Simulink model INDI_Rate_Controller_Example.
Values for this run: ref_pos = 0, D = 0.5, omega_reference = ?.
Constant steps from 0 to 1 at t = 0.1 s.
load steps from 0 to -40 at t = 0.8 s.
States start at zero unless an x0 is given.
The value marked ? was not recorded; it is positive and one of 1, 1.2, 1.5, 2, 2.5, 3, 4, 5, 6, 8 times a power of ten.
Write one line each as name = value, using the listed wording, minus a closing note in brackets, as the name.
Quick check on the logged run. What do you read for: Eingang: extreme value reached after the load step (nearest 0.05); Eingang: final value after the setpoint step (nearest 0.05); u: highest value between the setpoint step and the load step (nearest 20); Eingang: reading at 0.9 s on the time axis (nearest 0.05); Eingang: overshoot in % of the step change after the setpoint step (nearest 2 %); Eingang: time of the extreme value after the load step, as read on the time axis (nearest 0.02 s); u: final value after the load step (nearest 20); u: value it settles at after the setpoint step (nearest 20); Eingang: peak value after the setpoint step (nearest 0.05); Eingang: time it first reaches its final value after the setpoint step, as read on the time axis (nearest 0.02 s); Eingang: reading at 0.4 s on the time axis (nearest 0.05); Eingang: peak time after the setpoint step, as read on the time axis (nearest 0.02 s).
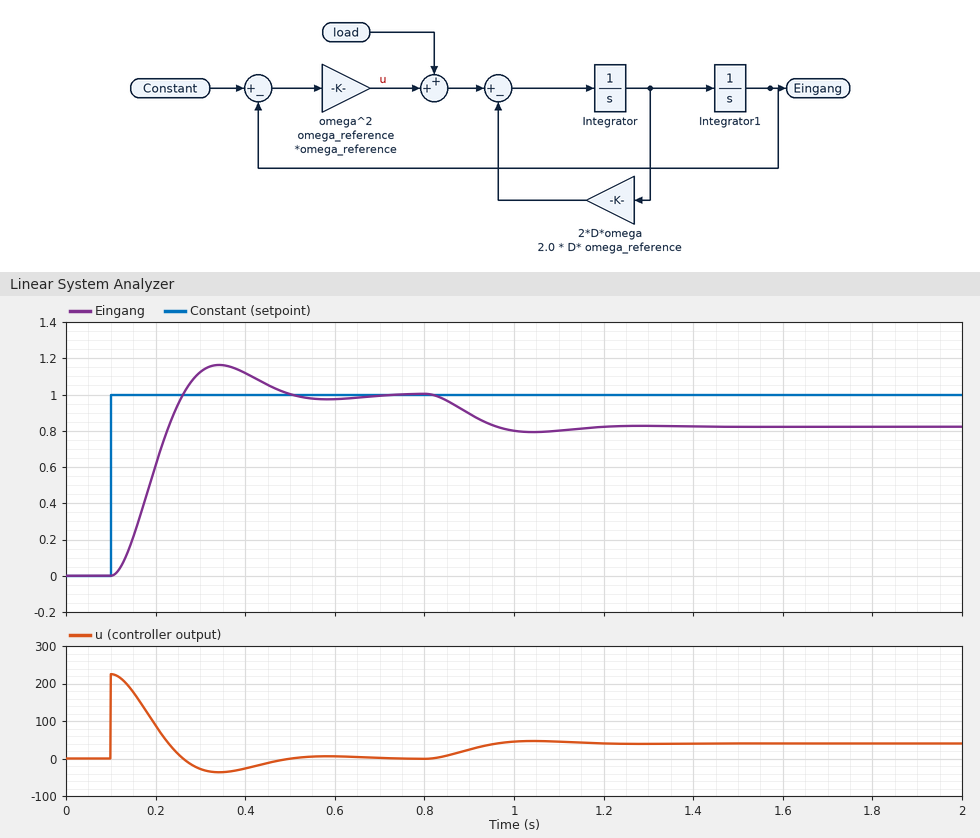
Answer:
Eingang: extreme value reached after the load step = 0.80
Eingang: final value after the setpoint step = 1.00
u: highest value between the setpoint step and the load step = 220
Eingang: reading at 0.9 s on the time axis = 0.90
Eingang: overshoot in % of the step change after the setpoint step = 16 %
Eingang: time of the extreme value after the load step, as read on the time axis = 1.04 s
u: final value after the load step = 40
u: value it settles at after the setpoint step = 0
Eingang: peak value after the setpoint step = 1.15
Eingang: time it first reaches its final value after the setpoint step, as read on the time axis = 0.26 s
Eingang: reading at 0.4 s on the time axis = 1.10
Eingang: peak time after the setpoint step, as read on the time axis = 0.34 s
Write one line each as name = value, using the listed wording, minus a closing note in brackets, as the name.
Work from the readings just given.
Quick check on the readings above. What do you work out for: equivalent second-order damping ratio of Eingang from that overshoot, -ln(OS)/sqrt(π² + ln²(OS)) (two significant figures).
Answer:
equivalent second-order damping ratio of Eingang from that overshoot, -ln(OS)/sqrt(π² + ln²(OS)) = 0.50
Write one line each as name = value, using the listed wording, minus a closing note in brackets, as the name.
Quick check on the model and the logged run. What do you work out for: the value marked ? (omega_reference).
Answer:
the value marked ? = 15
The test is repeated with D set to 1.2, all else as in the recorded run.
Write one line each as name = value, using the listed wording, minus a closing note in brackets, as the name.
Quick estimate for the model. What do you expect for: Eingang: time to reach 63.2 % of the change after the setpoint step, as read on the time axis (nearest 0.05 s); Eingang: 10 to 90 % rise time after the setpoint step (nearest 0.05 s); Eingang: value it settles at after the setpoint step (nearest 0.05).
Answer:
Eingang: time to reach 63.2 % of the change after the setpoint step, as read on the time axis = 0.25 s
Eingang: 10 to 90 % rise time after the setpoint step = 0.30 s
Eingang: value it settles at after the setpoint step = 1.00
